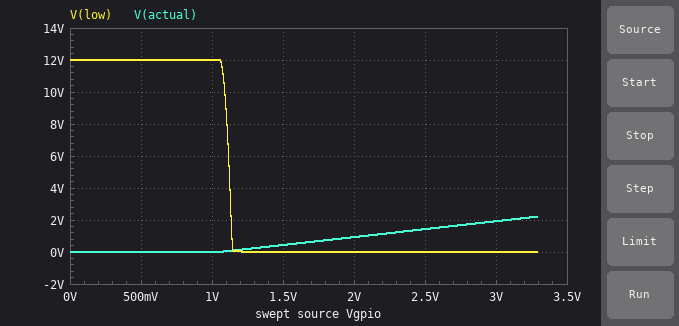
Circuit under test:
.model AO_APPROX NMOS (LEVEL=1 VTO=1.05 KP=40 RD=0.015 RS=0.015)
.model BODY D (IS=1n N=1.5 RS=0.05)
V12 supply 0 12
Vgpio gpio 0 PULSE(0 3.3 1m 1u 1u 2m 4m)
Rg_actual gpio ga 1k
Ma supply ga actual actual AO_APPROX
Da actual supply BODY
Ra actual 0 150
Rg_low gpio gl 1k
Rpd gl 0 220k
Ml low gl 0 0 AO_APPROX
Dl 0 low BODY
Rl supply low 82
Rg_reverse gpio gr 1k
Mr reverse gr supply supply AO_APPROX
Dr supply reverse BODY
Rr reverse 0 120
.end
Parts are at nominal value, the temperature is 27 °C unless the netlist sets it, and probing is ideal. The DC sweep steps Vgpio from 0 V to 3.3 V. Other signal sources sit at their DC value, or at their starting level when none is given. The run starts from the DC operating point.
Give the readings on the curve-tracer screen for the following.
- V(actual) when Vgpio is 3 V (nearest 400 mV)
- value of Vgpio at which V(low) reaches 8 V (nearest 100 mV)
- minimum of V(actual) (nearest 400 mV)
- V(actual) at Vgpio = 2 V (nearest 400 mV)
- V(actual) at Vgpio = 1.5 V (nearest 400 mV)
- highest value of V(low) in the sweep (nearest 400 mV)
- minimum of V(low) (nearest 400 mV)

2.0 V
1.1 V
0 V
800 mV
400 mV
12.0 V
0 V
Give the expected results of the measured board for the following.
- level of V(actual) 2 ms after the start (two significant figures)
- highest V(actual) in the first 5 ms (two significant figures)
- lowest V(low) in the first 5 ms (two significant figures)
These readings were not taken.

2.2 V
2.2 V
6.0 mV
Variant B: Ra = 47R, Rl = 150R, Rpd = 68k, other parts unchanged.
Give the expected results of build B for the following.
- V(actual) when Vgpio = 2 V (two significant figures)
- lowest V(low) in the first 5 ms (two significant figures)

920 mV
3.3 mV
